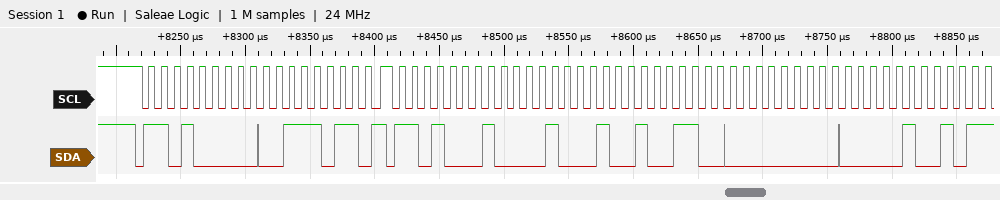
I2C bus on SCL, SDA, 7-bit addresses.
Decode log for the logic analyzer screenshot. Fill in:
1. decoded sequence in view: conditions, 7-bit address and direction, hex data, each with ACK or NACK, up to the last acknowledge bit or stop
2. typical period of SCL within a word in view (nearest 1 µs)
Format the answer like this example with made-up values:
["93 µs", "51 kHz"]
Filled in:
["start, address 68 write ACK, 3B ACK, repeated start, address 68 read ACK, 11 ACK, 4C ACK, 00 ACK, 09 ACK", "10 µs"]
